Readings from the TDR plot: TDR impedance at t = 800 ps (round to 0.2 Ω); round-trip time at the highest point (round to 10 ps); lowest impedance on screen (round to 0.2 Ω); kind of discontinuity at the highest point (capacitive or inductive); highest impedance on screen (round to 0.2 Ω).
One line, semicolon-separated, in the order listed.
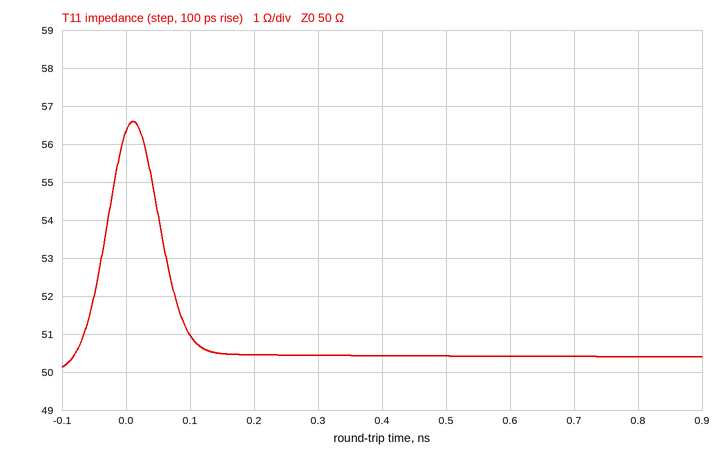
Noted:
50.4 Ω; 10 ps; 50.2 Ω; inductive; 56.6 Ω
